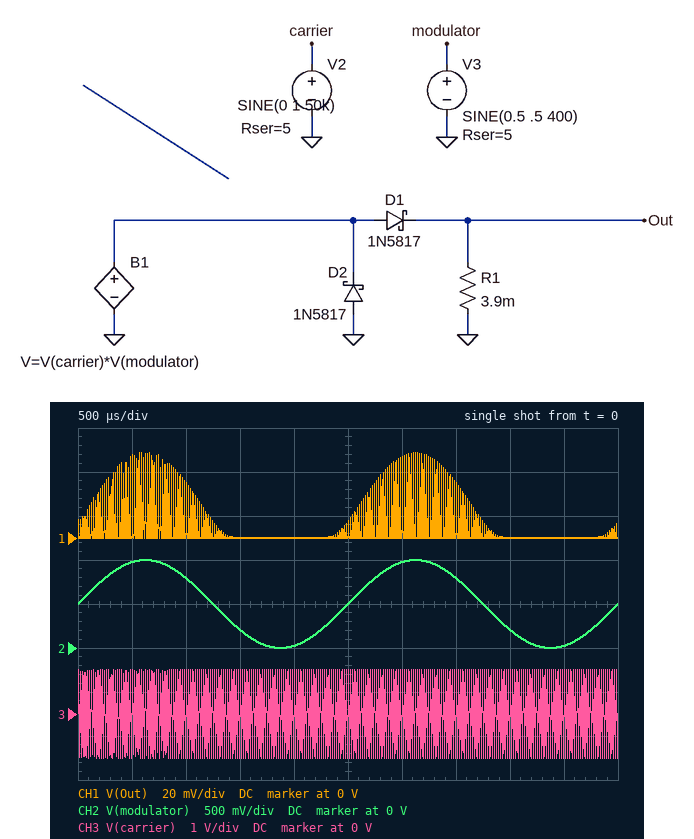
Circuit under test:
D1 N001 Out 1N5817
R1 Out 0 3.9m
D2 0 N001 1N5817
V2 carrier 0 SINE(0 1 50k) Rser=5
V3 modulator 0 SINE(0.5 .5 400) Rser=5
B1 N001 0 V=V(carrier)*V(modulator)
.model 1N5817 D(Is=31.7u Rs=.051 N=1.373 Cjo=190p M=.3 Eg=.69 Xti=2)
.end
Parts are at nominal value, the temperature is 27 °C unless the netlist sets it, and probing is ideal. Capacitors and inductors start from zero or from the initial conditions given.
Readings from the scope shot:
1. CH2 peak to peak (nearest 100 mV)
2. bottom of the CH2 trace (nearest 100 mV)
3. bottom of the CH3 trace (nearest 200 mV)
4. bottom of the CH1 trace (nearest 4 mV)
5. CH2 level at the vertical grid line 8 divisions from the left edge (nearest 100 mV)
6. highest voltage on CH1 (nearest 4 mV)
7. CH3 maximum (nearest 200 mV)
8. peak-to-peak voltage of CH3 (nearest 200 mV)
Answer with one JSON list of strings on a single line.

["1.0 V", "0 V", "-1.0 V", "0 V", "200 mV", "40 mV", "1.0 V", "2.0 V"]
